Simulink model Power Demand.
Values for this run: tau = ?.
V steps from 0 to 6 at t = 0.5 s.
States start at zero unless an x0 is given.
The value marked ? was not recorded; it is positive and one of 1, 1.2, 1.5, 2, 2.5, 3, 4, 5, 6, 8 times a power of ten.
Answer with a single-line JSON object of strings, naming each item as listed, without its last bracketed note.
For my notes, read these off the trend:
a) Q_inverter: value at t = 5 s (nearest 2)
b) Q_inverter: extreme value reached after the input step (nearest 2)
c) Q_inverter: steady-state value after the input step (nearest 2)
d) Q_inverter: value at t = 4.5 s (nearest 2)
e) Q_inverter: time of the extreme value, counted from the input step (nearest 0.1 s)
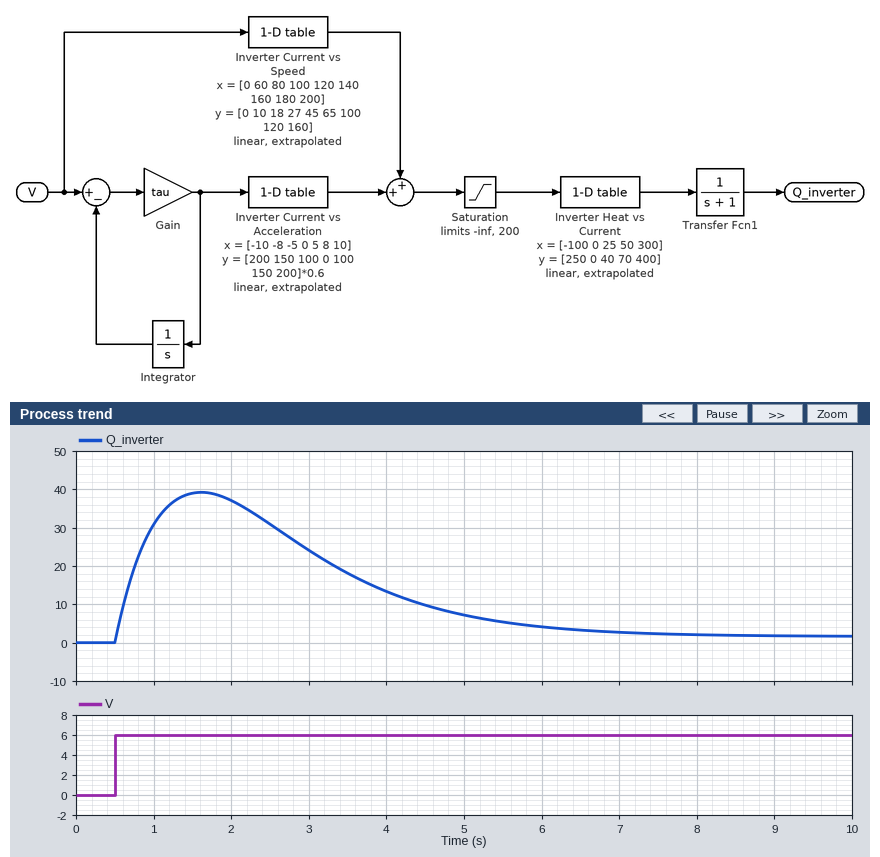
{"Q_inverter: value at t = 5 s": "8", "Q_inverter: extreme value reached after the input step": "40", "Q_inverter: steady-state value after the input step": "2", "Q_inverter: value at t = 4.5 s": "10", "Q_inverter: time of the extreme value, counted from the input step": "1.1 s"}
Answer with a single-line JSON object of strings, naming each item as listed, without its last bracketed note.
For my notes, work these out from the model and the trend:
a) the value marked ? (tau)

{"the value marked ?": "1"}
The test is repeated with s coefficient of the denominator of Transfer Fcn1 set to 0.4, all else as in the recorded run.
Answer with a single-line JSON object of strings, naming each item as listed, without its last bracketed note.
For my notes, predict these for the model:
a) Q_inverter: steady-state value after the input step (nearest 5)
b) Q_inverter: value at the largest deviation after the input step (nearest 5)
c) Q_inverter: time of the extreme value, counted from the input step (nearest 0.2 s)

{"Q_inverter: steady-state value after the input step": "0", "Q_inverter: value at the largest deviation after the input step": "55", "Q_inverter: time of the extreme value, counted from the input step": "0.6 s"}
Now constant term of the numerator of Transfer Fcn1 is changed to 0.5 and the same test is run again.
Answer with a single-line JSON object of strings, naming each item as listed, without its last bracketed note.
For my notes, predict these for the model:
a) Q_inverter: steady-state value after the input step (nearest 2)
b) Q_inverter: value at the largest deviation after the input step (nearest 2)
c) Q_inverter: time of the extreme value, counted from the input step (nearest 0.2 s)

{"Q_inverter: steady-state value after the input step": "0", "Q_inverter: value at the largest deviation after the input step": "20", "Q_inverter: time of the extreme value, counted from the input step": "1.2 s"}
